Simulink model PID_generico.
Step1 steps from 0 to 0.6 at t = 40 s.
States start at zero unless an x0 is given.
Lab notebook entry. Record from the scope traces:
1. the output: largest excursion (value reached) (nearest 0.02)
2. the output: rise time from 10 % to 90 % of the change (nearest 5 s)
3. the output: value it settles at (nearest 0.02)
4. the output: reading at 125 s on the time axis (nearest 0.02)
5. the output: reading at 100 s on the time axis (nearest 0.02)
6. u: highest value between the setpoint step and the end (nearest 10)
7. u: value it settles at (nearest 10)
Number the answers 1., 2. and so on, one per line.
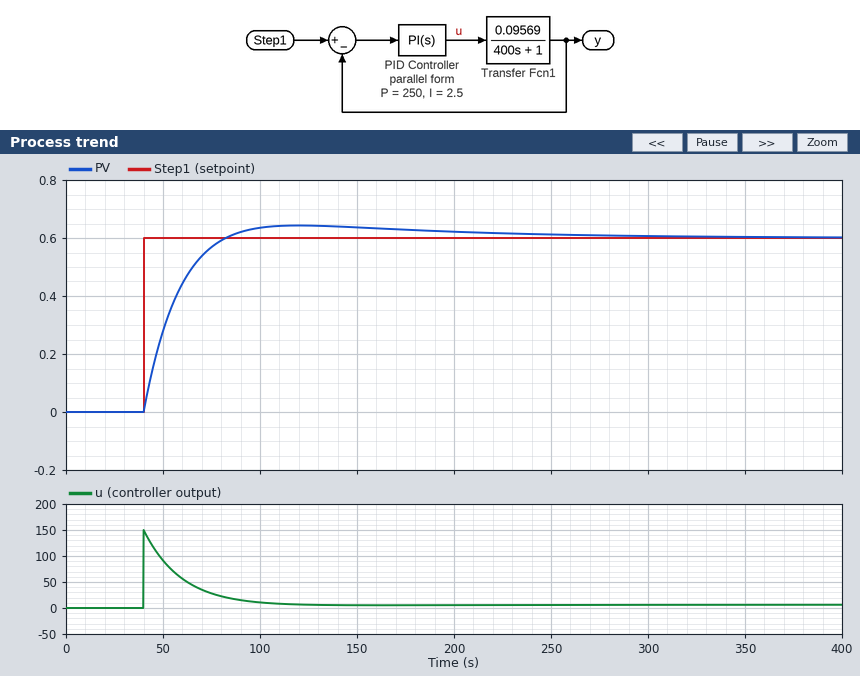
1. 0.64
2. 30 s
3. 0.60
4. 0.64
5. 0.64
6. 150
7. 10
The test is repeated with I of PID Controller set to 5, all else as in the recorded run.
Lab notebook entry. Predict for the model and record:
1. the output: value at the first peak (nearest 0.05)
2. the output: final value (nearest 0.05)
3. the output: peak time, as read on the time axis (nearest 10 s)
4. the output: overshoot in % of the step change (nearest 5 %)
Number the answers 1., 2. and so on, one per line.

1. 0.70
2. 0.60
3. 100 s
4. 15 %
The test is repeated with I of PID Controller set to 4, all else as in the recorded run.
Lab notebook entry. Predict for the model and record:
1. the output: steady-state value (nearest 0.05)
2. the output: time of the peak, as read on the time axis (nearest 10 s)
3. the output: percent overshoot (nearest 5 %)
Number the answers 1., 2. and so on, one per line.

1. 0.60
2. 110 s
3. 10 %
